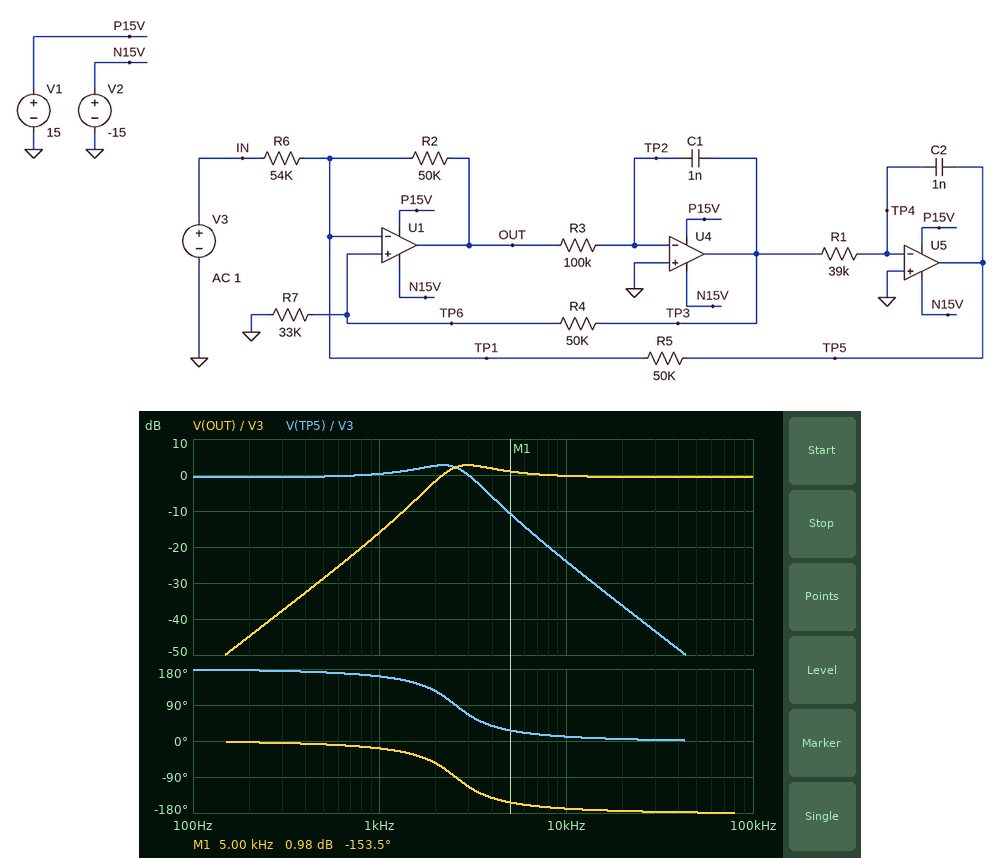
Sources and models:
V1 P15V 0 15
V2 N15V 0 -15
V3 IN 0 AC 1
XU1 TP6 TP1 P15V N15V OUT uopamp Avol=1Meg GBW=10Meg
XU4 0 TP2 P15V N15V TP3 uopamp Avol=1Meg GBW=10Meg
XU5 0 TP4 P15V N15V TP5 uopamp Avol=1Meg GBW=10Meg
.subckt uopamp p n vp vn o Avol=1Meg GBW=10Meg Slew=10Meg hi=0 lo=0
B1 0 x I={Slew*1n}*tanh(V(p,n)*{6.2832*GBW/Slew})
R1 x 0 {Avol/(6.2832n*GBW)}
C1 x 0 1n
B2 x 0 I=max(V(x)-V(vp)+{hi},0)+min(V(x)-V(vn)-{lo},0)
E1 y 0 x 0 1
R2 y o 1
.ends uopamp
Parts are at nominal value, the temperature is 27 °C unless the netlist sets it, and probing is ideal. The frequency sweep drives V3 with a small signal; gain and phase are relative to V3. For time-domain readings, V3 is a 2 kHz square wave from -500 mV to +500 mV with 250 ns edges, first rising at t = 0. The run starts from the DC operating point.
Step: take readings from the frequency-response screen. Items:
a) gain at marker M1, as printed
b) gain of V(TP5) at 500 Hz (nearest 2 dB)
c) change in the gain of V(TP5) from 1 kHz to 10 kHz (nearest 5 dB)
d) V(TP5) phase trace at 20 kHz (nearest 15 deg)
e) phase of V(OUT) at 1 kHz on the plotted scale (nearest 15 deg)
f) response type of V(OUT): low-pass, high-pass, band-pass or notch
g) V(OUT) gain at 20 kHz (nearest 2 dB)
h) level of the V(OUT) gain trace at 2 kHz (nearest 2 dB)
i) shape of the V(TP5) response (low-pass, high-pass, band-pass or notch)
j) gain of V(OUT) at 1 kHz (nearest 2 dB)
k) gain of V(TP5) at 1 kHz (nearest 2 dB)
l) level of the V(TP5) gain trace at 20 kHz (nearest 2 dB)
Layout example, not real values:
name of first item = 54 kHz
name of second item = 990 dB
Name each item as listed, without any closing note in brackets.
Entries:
gain at marker M1, as printed = 0.98 dB
gain of V(TP5) at 500 Hz = 0 dB
change in the gain of V(TP5) from 1 kHz to 10 kHz = -25 dB
V(TP5) phase trace at 20 kHz = 0 deg
phase of V(OUT) at 1 kHz on the plotted scale = -15 deg
response type of V(OUT): low-pass, high-pass, band-pass or notch = high-pass
V(OUT) gain at 20 kHz = 0 dB
level of the V(OUT) gain trace at 2 kHz = -2 dB
shape of the V(TP5) response = low-pass
gain of V(OUT) at 1 kHz = -16 dB
gain of V(TP5) at 1 kHz = 0 dB
level of the V(TP5) gain trace at 20 kHz = -36 dB
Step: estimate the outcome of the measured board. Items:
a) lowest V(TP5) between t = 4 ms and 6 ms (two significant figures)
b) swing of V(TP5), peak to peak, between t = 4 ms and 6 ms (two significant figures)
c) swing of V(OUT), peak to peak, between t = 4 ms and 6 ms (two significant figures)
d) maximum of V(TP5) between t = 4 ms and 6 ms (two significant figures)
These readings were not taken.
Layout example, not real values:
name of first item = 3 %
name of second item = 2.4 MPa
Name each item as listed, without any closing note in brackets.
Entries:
lowest V(TP5) between t = 4 ms and 6 ms = -820 mV
swing of V(TP5), peak to peak, between t = 4 ms and 6 ms = 1.6 V
swing of V(OUT), peak to peak, between t = 4 ms and 6 ms = 2.1 V
maximum of V(TP5) between t = 4 ms and 6 ms = 820 mV
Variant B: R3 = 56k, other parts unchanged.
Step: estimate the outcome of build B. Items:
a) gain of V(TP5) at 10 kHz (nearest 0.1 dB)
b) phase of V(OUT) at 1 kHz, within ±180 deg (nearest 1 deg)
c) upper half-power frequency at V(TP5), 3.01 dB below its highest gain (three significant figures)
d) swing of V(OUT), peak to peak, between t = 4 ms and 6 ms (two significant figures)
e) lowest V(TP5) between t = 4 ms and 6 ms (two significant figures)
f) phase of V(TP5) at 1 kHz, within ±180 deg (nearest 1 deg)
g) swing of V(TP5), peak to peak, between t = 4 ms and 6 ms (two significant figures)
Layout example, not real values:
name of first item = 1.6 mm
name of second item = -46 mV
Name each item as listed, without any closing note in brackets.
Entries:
gain of V(TP5) at 10 kHz = -18.9 dB
phase of V(OUT) at 1 kHz, within ±180 deg = -17 deg
upper half-power frequency at V(TP5), 3.01 dB below its highest gain = 4.00 kHz
swing of V(OUT), peak to peak, between t = 4 ms and 6 ms = 1.8 V
lowest V(TP5) between t = 4 ms and 6 ms = -630 mV
phase of V(TP5) at 1 kHz, within ±180 deg = 163 deg
swing of V(TP5), peak to peak, between t = 4 ms and 6 ms = 1.3 V
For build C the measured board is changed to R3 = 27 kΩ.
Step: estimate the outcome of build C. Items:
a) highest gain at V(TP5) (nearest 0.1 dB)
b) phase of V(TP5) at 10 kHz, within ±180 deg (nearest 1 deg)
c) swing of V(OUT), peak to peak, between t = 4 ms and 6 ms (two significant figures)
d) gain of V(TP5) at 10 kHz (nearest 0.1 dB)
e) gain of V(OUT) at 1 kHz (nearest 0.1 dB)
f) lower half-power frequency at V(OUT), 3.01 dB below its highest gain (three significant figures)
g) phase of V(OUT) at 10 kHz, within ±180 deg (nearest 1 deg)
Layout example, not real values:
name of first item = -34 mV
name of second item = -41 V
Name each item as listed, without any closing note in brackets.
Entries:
highest gain at V(TP5) = -0.7 dB
phase of V(TP5) at 10 kHz, within ±180 deg = 42 deg
swing of V(OUT), peak to peak, between t = 4 ms and 6 ms = 1.8 V
gain of V(TP5) at 10 kHz = -13.2 dB
gain of V(OUT) at 1 kHz = -28.3 dB
lower half-power frequency at V(OUT), 3.01 dB below its highest gain = 4.85 kHz
phase of V(OUT) at 10 kHz, within ±180 deg = -138 deg
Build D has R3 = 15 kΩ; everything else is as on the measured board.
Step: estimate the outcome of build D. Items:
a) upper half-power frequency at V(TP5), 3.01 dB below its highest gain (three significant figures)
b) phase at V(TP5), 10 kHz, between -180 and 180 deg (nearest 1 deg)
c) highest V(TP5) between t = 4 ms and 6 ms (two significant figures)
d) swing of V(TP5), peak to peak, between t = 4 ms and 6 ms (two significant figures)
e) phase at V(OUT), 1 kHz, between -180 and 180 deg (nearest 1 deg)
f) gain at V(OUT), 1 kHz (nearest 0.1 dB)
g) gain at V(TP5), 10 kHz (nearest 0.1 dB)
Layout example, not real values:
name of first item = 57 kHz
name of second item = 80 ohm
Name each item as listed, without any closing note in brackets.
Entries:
upper half-power frequency at V(TP5), 3.01 dB below its highest gain = 4.64 kHz
phase at V(TP5), 10 kHz, between -180 and 180 deg = 65 deg
highest V(TP5) between t = 4 ms and 6 ms = 460 mV
swing of V(TP5), peak to peak, between t = 4 ms and 6 ms = 930 mV
phase at V(OUT), 1 kHz, between -180 and 180 deg = -16 deg
gain at V(OUT), 1 kHz = -33.5 dB
gain at V(TP5), 10 kHz = -10.6 dB
